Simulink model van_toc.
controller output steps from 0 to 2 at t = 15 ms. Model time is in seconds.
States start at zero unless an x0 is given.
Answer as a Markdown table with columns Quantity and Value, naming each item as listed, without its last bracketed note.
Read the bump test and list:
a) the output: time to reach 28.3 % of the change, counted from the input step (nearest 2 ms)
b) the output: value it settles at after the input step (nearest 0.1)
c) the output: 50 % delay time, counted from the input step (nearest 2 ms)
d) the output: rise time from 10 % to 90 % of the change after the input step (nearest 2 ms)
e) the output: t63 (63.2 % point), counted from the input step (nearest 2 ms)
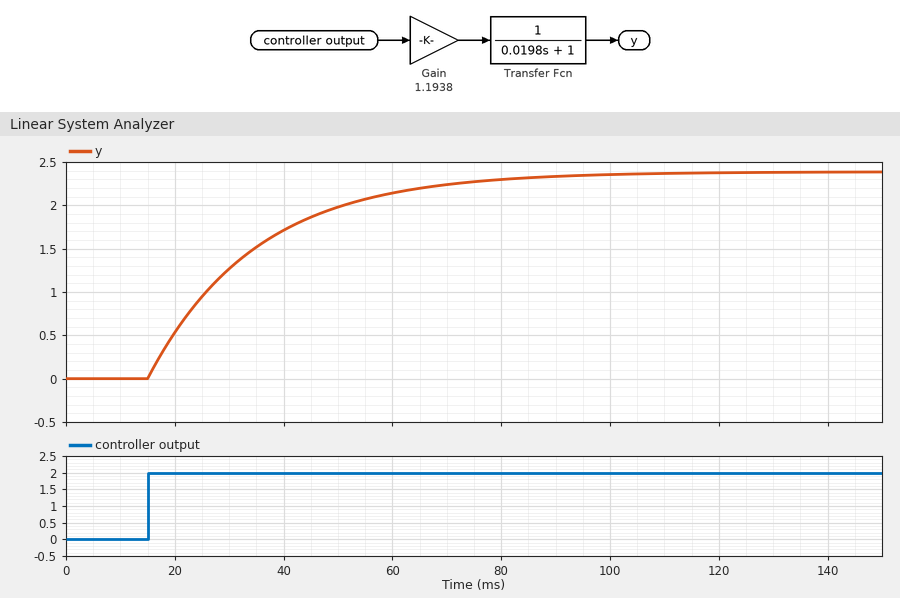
| Quantity | Value |
|---|---|
| the output: time to reach 28.3 % of the change, counted from the input step | 6 ms |
| the output: value it settles at after the input step | 2.4 |
| the output: 50 % delay time, counted from the input step | 14 ms |
| the output: rise time from 10 % to 90 % of the change after the input step | 44 ms |
| the output: t63 (63.2 % point), counted from the input step | 20 ms |
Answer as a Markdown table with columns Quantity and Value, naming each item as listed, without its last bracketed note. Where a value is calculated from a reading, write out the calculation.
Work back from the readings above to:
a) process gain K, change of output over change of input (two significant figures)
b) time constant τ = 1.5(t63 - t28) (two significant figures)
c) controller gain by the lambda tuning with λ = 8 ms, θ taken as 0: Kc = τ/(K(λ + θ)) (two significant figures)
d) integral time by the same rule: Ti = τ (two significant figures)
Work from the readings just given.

| Quantity | Value |
|---|---|
| process gain K, change of output over change of input | (2.4 - 0) / 2 = 1.2 |
| time constant τ = 1.5(t63 - t28) | 1.5 × (20 - 6) = 21 ms |
| controller gain by the lambda tuning with λ = 8 ms, θ taken as 0: Kc = τ/(K(λ + θ)) | 21 / (1.2 × (8 + 0)) = 2.2 |
| integral time by the same rule: Ti = τ | 21 ms |
